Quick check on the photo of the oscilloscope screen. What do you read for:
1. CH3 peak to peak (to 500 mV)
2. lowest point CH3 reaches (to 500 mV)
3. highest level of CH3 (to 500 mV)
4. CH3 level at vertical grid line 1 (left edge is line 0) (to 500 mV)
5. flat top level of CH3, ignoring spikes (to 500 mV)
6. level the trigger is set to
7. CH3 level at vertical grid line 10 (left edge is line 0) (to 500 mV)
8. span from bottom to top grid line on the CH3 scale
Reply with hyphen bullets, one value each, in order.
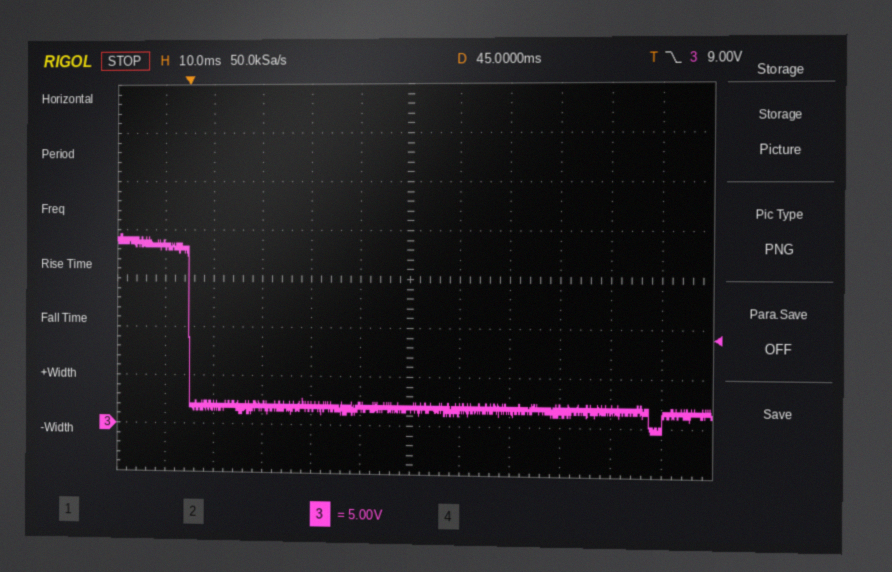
- 20.0 V
- -500 mV
- 19.5 V
- 18.5 V
- 18.5 V
- 9.00 V
- 2.0 V
- 40 V
